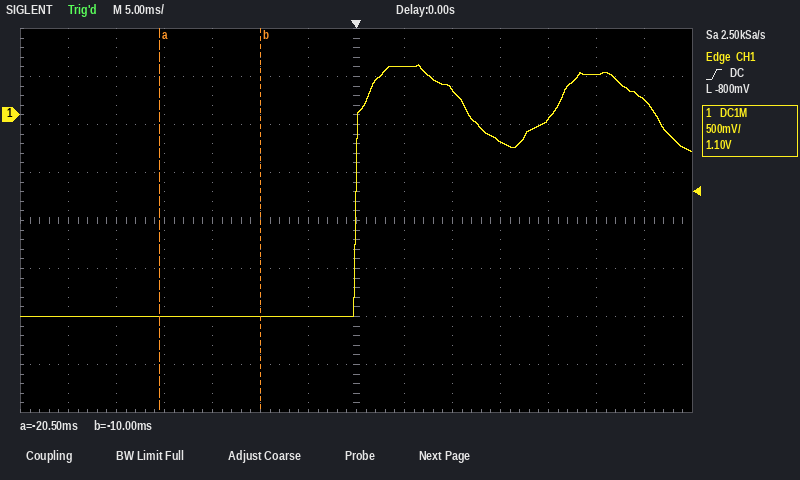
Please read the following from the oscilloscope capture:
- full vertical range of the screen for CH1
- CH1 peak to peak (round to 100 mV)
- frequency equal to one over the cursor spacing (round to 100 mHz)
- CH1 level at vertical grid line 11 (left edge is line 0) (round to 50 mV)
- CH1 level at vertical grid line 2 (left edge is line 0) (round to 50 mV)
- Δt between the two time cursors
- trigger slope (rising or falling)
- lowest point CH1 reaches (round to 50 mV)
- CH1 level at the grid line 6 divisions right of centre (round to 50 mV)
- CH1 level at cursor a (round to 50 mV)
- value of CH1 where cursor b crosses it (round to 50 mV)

4 V
2.60 V
95.2 Hz
-50 mV
-2.10 V
10.5 ms
rising
-2.10 V
150 mV
-2.10 V
-2.10 V
